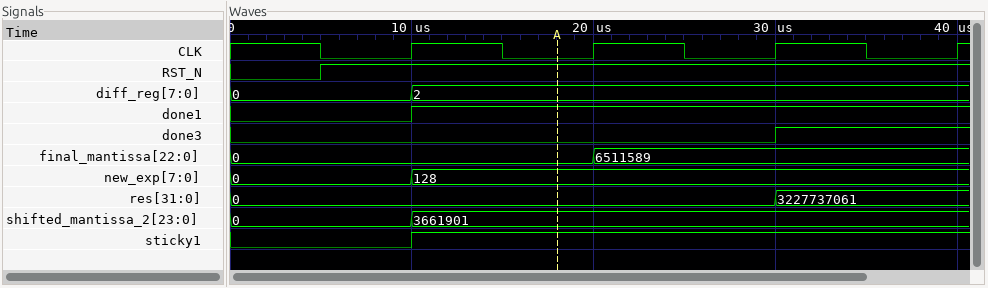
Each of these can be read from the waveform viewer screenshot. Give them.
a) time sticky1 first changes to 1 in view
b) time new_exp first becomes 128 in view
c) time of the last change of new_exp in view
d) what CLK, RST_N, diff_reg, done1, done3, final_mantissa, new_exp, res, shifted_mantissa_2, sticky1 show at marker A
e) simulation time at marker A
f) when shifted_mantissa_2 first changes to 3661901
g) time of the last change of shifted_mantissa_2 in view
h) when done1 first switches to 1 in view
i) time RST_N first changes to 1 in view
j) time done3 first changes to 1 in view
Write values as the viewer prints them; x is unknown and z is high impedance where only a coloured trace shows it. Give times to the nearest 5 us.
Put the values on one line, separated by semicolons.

10 us; 10 us; 10 us; CLK=0, RST_N=1, diff_reg=2, done1=1, done3=0, final_mantissa=0, new_exp=128, res=0, shifted_mantissa_2=3661901, sticky1=1; 20 us; 10 us; 10 us; 10 us; 5 us; 30 us
